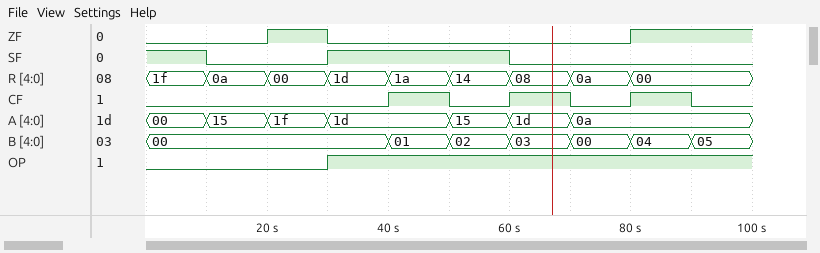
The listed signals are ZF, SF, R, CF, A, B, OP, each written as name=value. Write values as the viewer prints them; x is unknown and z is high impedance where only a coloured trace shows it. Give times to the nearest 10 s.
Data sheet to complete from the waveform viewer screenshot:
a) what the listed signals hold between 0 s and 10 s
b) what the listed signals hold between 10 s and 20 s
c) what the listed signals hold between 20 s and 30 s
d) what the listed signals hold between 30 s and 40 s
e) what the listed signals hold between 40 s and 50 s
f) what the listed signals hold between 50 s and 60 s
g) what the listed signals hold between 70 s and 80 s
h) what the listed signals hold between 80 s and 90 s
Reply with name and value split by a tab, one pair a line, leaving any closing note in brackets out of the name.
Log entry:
what the listed signals hold between 0 s and 10 s	ZF=0, SF=1, R=1f, CF=0, A=00, B=00, OP=0
what the listed signals hold between 10 s and 20 s	ZF=0, SF=0, R=0a, CF=0, A=15, B=00, OP=0
what the listed signals hold between 20 s and 30 s	ZF=1, SF=0, R=00, CF=0, A=1f, B=00, OP=0
what the listed signals hold between 30 s and 40 s	ZF=0, SF=1, R=1d, CF=0, A=1d, B=00, OP=1
what the listed signals hold between 40 s and 50 s	ZF=0, SF=1, R=1a, CF=1, A=1d, B=01, OP=1
what the listed signals hold between 50 s and 60 s	ZF=0, SF=1, R=14, CF=0, A=15, B=02, OP=1
what the listed signals hold between 70 s and 80 s	ZF=0, SF=0, R=0a, CF=0, A=0a, B=00, OP=1
what the listed signals hold between 80 s and 90 s	ZF=1, SF=0, R=00, CF=1, A=0a, B=04, OP=1
